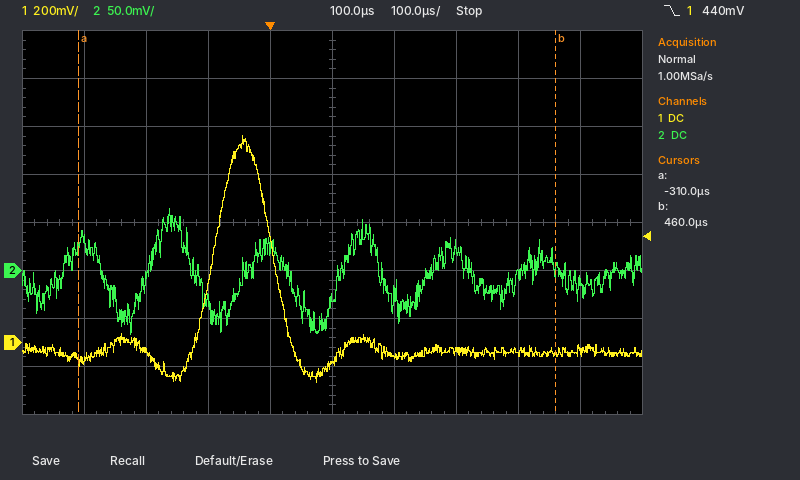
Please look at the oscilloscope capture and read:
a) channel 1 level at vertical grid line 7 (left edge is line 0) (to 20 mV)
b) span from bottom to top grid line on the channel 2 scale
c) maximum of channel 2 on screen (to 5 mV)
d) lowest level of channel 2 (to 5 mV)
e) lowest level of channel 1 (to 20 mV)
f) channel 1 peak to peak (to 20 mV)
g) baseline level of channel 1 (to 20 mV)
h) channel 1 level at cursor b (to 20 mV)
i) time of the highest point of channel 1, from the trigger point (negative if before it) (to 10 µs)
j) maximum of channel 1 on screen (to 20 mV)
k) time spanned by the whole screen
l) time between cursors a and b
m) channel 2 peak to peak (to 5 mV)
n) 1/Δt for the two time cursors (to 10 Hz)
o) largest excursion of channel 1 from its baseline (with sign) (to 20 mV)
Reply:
-40 mV
400 mV
65 mV
-65 mV
-160 mV
1.02 V
-40 mV
-40 mV
-40 µs
860 mV
1 ms
770 µs
130 mV
1.30 kHz
+900 mV
